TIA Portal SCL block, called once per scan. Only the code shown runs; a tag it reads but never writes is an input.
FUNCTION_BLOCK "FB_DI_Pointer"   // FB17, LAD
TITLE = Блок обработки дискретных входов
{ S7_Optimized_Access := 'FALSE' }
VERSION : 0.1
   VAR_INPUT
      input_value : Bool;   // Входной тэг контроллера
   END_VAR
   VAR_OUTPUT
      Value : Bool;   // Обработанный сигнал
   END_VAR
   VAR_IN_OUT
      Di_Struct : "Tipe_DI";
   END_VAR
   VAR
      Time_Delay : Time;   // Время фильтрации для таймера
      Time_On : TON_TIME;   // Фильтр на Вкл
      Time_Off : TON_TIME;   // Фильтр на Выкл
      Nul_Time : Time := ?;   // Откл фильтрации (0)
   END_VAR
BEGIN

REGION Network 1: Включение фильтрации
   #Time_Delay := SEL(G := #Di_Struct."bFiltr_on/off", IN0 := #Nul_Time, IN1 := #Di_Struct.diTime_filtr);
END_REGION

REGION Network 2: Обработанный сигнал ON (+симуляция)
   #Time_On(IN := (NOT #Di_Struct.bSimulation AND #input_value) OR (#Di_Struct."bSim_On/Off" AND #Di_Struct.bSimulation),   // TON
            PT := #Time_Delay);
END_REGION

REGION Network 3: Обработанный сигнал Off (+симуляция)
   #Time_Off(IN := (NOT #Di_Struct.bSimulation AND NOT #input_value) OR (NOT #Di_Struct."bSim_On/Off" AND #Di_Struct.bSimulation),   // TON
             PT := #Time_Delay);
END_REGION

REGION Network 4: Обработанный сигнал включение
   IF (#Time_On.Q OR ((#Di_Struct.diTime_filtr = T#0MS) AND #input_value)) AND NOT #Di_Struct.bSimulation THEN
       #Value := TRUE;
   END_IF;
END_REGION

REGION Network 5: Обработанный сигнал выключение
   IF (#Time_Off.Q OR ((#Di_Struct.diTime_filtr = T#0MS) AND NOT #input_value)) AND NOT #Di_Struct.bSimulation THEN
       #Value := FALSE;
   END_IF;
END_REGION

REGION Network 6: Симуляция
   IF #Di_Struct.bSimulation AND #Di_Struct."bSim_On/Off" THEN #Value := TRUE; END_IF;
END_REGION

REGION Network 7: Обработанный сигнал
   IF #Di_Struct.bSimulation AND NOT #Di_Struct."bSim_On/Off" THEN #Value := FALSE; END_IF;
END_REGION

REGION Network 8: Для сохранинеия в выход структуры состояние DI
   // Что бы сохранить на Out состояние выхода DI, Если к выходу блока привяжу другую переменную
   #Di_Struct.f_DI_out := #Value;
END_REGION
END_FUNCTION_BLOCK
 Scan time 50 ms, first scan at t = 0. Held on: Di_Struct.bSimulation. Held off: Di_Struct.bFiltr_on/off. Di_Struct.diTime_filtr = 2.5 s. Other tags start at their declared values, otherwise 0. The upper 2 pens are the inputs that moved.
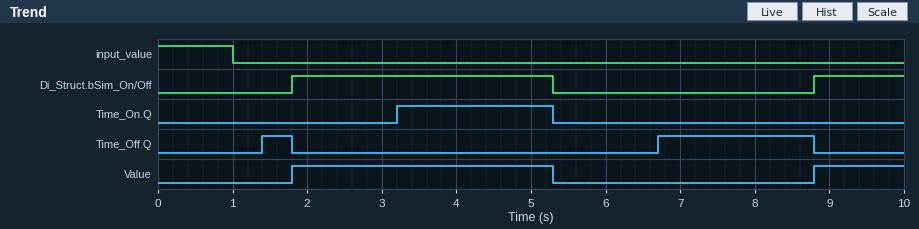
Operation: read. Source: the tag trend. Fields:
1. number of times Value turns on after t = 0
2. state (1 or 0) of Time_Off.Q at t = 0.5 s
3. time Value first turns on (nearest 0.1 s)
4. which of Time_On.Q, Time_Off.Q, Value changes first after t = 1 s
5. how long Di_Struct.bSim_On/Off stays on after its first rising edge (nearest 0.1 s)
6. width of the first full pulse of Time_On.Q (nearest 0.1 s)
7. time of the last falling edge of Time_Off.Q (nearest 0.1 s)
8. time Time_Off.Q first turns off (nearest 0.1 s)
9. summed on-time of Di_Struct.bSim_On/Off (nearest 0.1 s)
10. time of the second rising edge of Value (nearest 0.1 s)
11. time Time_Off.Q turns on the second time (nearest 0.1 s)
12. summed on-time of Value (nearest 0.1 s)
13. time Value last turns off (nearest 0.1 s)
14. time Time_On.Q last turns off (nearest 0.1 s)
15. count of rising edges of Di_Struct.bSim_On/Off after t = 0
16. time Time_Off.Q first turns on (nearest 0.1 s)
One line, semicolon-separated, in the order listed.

2; 0; 1.8 s; Time_Off.Q; 3.5 s; 2.1 s; 8.8 s; 1.8 s; 4.7 s; 8.8 s; 6.7 s; 4.7 s; 5.3 s; 5.3 s; 2; 1.4 s
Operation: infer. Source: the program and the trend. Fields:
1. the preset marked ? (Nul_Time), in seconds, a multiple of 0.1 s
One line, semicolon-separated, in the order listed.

1.4 s
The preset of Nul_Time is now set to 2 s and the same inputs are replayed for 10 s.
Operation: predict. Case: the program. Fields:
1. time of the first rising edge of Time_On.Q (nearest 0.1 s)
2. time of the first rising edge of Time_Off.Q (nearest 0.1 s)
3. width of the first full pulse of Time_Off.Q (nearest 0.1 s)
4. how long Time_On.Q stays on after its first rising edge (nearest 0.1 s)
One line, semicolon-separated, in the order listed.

3.8 s; 7.3 s; 1.5 s; 1.5 s
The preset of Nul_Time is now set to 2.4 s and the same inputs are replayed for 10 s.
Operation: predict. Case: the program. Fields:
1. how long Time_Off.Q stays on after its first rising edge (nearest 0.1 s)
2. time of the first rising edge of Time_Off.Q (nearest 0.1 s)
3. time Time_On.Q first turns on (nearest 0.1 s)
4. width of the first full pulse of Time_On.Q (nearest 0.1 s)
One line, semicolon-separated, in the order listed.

1.1 s; 7.7 s; 4.2 s; 1.1 s
